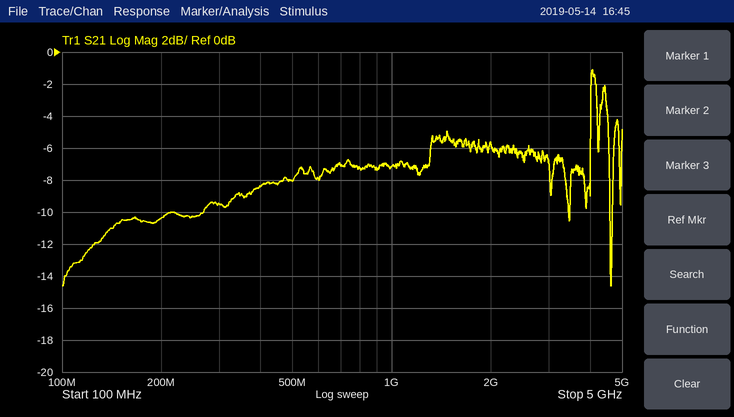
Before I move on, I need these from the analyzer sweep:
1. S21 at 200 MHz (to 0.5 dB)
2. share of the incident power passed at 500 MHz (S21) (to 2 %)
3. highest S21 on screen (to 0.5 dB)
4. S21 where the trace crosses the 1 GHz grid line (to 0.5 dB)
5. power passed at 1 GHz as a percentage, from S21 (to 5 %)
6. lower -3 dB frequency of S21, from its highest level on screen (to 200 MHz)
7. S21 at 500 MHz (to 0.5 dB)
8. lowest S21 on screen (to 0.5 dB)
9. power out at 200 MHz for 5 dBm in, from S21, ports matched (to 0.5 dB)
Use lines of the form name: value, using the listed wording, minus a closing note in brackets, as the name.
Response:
S21 at 200 MHz: -10.5 dB
share of the incident power passed at 500 MHz (S21): 16 %
highest S21 on screen: -1.0 dB
S21 where the trace crosses the 1 GHz grid line: -7.0 dB
power passed at 1 GHz as a percentage, from S21: 20 %
lower -3 dB frequency of S21, from its highest level on screen: 4.0 GHz
S21 at 500 MHz: -8.0 dB
lowest S21 on screen: -14.5 dB
power out at 200 MHz for 5 dBm in, from S21, ports matched: -5.5 dBm
